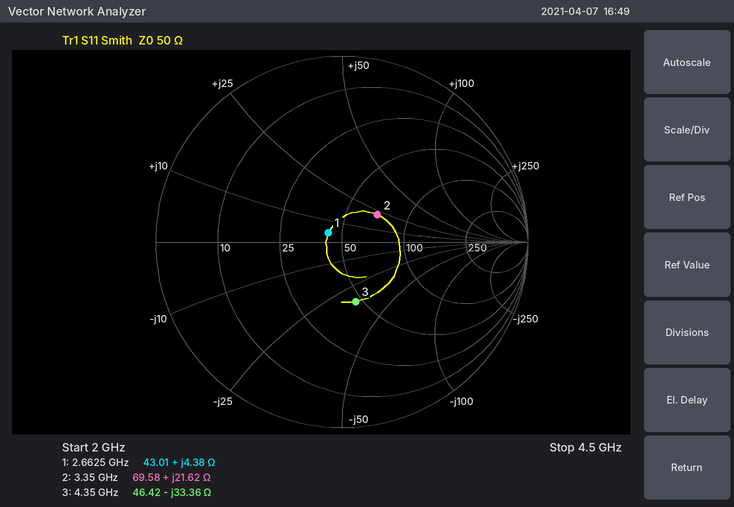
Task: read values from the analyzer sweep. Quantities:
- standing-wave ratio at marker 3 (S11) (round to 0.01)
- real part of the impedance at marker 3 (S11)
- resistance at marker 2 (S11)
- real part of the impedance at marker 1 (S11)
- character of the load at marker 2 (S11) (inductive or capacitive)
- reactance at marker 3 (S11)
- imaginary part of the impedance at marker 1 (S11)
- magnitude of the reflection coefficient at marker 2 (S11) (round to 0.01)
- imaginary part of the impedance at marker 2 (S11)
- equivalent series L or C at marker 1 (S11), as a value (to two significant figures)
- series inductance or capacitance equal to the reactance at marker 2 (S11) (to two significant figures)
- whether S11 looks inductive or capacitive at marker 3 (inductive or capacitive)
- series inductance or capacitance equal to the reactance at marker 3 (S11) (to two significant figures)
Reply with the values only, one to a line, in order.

1.98
46.42 Ω
69.58 Ω
43.01 Ω
inductive
-33.36 Ω
+4.38 Ω
0.24
+21.62 Ω
260 pH
1.0 nH
capacitive
1.1 pF
